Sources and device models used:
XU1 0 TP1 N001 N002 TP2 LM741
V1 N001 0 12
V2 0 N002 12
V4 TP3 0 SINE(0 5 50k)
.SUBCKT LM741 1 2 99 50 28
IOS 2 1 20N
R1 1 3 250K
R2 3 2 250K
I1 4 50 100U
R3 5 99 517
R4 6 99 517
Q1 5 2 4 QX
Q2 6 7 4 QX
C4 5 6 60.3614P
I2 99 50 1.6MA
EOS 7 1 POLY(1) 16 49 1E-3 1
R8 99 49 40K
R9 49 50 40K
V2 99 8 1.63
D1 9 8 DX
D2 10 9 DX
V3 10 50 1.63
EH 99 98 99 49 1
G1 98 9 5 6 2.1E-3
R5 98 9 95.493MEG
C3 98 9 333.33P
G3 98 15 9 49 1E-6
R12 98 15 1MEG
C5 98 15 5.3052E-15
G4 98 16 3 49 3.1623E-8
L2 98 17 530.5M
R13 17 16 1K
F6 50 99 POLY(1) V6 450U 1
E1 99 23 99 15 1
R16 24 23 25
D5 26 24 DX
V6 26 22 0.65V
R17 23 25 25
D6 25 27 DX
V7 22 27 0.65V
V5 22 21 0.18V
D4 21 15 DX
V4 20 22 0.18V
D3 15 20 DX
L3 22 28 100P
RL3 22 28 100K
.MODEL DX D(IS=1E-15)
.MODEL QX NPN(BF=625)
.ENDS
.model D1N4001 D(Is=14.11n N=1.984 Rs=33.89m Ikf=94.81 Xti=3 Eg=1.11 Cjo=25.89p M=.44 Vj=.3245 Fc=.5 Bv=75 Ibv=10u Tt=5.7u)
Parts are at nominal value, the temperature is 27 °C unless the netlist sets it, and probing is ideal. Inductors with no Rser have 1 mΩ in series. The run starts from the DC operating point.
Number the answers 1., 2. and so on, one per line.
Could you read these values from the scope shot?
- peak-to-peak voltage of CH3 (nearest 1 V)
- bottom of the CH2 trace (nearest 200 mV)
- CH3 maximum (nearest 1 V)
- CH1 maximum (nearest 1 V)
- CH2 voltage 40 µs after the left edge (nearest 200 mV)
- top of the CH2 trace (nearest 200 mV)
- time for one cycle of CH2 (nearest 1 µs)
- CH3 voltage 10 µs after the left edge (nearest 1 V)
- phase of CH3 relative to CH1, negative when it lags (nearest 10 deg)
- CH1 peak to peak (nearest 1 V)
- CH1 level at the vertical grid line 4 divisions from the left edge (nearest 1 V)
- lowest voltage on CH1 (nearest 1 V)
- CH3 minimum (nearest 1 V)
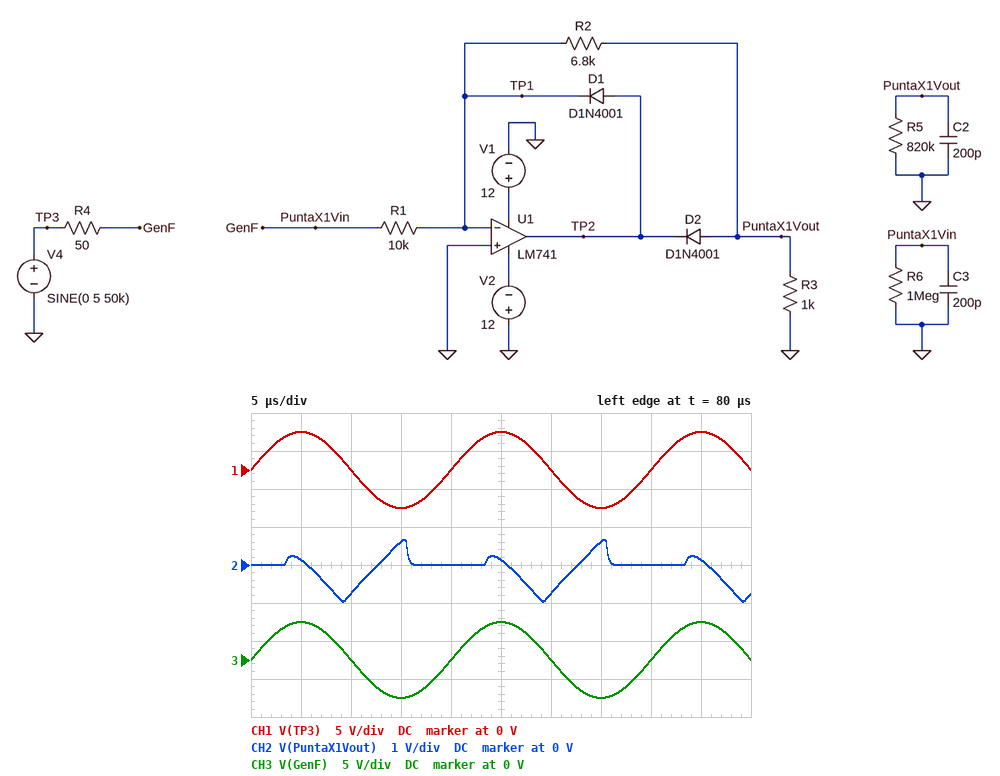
1. 10 V
2. -1.0 V
3. 5 V
4. 5 V
5. 0 V
6. 600 mV
7. 20 µs
8. 0 V
9. 0 deg
10. 10 V
11. 0 V
12. -5 V
13. -5 V
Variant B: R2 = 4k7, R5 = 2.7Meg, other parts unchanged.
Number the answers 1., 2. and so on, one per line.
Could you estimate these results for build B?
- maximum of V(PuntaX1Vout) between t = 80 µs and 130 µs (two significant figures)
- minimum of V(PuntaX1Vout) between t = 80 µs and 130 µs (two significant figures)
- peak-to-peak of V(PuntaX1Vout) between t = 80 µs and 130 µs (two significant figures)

1. 600 mV
2. -870 mV
3. 1.5 V
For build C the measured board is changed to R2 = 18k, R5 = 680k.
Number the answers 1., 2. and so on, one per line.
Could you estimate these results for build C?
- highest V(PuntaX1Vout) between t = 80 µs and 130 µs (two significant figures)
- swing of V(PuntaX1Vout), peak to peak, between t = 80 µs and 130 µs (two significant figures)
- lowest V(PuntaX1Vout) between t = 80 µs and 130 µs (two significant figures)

1. 770 mV
2. 1.9 V
3. -1.1 V
